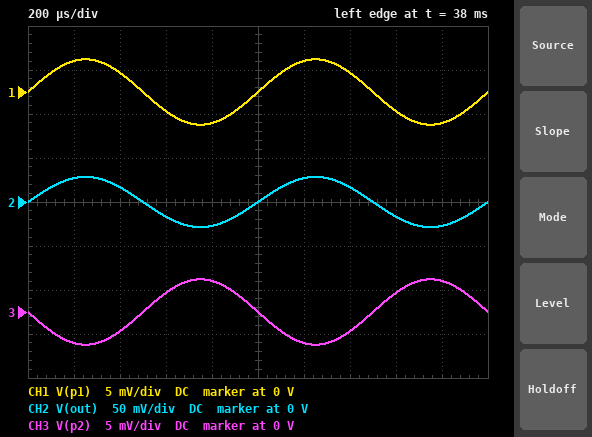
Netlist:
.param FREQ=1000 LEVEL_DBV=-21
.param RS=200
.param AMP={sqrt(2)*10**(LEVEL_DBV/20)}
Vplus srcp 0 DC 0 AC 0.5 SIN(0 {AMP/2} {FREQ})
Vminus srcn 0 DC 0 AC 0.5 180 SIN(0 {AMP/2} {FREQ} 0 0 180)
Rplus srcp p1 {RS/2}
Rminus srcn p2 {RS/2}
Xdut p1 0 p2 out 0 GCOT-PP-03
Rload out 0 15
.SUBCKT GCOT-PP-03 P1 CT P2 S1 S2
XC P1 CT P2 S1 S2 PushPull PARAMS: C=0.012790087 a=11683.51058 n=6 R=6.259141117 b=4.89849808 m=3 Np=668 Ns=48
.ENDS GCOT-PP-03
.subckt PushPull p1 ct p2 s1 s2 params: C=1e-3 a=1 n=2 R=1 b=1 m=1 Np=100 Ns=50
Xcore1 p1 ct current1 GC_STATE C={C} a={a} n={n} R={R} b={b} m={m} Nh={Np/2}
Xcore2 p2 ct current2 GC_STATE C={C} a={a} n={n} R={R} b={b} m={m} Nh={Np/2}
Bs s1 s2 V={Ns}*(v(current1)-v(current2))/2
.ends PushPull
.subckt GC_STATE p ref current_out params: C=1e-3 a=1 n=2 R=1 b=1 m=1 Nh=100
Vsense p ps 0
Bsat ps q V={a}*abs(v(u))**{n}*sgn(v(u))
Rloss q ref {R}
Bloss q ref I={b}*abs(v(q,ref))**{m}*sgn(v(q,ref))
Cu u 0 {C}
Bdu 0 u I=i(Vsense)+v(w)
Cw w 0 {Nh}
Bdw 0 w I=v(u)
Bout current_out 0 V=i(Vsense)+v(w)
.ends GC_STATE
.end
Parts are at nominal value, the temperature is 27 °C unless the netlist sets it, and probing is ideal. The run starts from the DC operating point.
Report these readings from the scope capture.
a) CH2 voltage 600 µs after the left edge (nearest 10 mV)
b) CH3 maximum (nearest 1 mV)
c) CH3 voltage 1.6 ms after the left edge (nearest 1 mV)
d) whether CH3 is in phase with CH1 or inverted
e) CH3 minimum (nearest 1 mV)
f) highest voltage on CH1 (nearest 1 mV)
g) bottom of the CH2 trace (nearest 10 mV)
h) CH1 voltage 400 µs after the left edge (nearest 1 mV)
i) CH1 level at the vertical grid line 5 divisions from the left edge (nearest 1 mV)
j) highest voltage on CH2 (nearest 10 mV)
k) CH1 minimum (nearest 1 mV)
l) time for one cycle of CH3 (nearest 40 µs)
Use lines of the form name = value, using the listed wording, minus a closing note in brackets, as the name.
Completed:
CH2 voltage 600 µs after the left edge = -20 mV
CH3 maximum = 4 mV
CH3 voltage 1.6 ms after the left edge = 2 mV
whether CH3 is in phase with CH1 or inverted = inverted
CH3 minimum = -4 mV
highest voltage on CH1 = 4 mV
bottom of the CH2 trace = -30 mV
CH1 voltage 400 µs after the left edge = 2 mV
CH1 level at the vertical grid line 5 divisions from the left edge = 0 V
highest voltage on CH2 = 30 mV
CH1 minimum = -4 mV
time for one cycle of CH3 = 1.00 ms
